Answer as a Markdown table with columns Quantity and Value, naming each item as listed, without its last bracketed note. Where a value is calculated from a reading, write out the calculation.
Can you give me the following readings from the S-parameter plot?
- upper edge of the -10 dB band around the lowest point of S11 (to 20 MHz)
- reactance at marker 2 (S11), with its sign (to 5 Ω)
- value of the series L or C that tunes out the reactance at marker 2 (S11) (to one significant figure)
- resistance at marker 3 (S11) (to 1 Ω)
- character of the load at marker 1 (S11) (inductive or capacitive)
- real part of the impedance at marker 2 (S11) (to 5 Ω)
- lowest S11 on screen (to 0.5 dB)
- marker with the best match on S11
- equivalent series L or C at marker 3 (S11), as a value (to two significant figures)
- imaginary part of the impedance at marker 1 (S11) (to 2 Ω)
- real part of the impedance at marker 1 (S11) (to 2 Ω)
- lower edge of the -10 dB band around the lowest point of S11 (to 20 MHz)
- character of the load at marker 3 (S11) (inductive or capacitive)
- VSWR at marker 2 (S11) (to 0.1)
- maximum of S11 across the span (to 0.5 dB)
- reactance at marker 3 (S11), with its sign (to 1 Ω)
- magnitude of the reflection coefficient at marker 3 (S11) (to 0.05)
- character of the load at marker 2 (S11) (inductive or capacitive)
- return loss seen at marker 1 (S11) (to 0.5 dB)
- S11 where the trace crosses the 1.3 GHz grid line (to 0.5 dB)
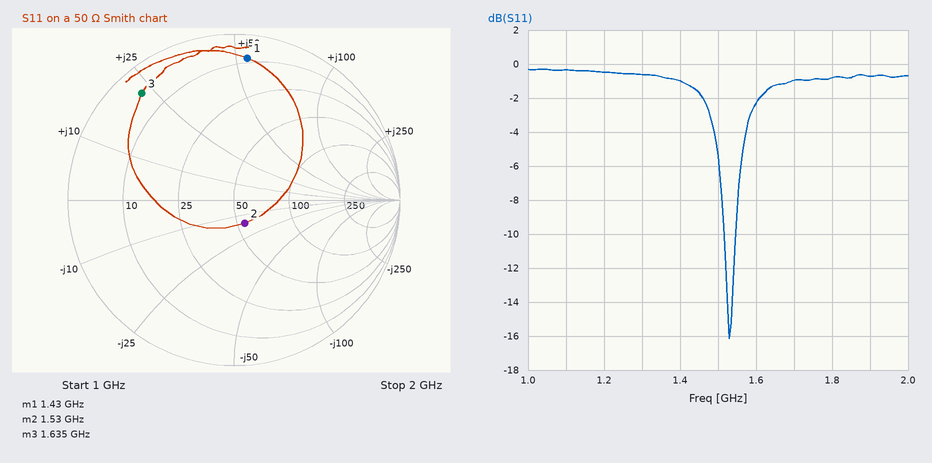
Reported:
| Quantity | Value |
|---|---|
| upper edge of the -10 dB band around the lowest point of S11 | 1.54 GHz |
| reactance at marker 2 (S11), with its sign | -15 Ω |
| value of the series L or C that tunes out the reactance at marker 2 (S11) | L = 15 Ω/(2π × 1.53 GHz) ≈ 2 nH |
| resistance at marker 3 (S11) | 5 Ω |
| character of the load at marker 1 (S11) | inductive |
| real part of the impedance at marker 2 (S11) | 55 Ω |
| lowest S11 on screen | -16.0 dB |
| marker with the best match on S11 | marker 2 |
| equivalent series L or C at marker 3 (S11), as a value | L = 23 Ω/(2π × 1.635 GHz) ≈ 2.2 nH |
| imaginary part of the impedance at marker 1 (S11) | +54 Ω |
| real part of the impedance at marker 1 (S11) | 8 Ω |
| lower edge of the -10 dB band around the lowest point of S11 | 1.52 GHz |
| character of the load at marker 3 (S11) | inductive |
| VSWR at marker 2 (S11) | 1.4 |
| maximum of S11 across the span | -0.5 dB |
| reactance at marker 3 (S11), with its sign | +23 Ω |
| magnitude of the reflection coefficient at marker 3 (S11) | 0.85 |
| character of the load at marker 2 (S11) | capacitive |
| return loss seen at marker 1 (S11) | 1.5 dB |
| S11 where the trace crosses the 1.3 GHz grid line | -0.5 dB |
